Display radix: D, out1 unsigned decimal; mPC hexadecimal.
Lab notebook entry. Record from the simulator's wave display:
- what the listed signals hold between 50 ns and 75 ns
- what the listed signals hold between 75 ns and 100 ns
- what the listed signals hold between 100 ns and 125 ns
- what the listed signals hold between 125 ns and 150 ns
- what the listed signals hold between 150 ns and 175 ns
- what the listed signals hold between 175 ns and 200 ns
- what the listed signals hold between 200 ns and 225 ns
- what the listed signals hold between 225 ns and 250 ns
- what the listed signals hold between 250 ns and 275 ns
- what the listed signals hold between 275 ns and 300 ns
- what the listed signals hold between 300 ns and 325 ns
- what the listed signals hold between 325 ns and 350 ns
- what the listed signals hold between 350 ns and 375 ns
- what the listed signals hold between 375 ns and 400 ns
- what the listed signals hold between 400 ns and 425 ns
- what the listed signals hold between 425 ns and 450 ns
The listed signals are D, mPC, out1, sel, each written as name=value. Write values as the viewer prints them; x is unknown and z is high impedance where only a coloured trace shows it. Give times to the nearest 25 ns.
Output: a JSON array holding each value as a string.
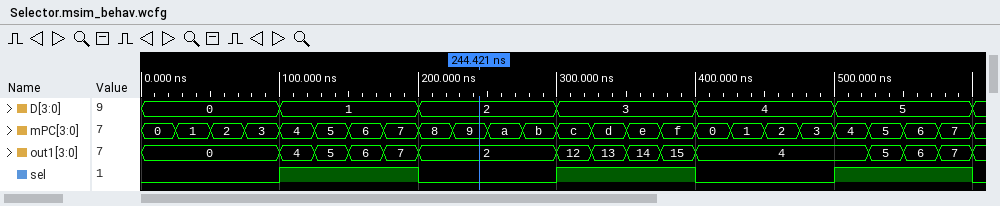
["D=0, mPC=2, out1=0, sel=0", "D=0, mPC=3, out1=0, sel=0", "D=1, mPC=4, out1=4, sel=1", "D=1, mPC=5, out1=5, sel=1", "D=1, mPC=6, out1=6, sel=1", "D=1, mPC=7, out1=7, sel=1", "D=2, mPC=8, out1=2, sel=0", "D=2, mPC=9, out1=2, sel=0", "D=2, mPC=a, out1=2, sel=0", "D=2, mPC=b, out1=2, sel=0", "D=3, mPC=c, out1=12, sel=1", "D=3, mPC=d, out1=13, sel=1", "D=3, mPC=e, out1=14, sel=1", "D=3, mPC=f, out1=15, sel=1", "D=4, mPC=0, out1=4, sel=0", "D=4, mPC=1, out1=4, sel=0"]
